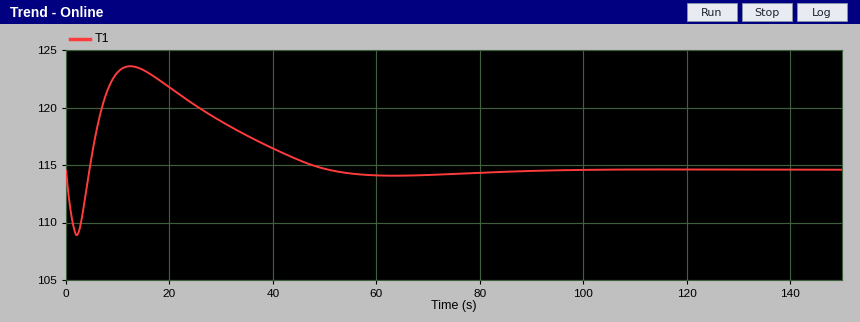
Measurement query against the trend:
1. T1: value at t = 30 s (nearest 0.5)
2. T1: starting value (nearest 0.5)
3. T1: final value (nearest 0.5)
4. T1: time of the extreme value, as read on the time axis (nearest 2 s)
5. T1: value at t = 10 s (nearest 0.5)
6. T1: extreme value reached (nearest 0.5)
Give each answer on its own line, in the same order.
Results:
119.0
114.5
114.5
12 s
123.0
123.5
